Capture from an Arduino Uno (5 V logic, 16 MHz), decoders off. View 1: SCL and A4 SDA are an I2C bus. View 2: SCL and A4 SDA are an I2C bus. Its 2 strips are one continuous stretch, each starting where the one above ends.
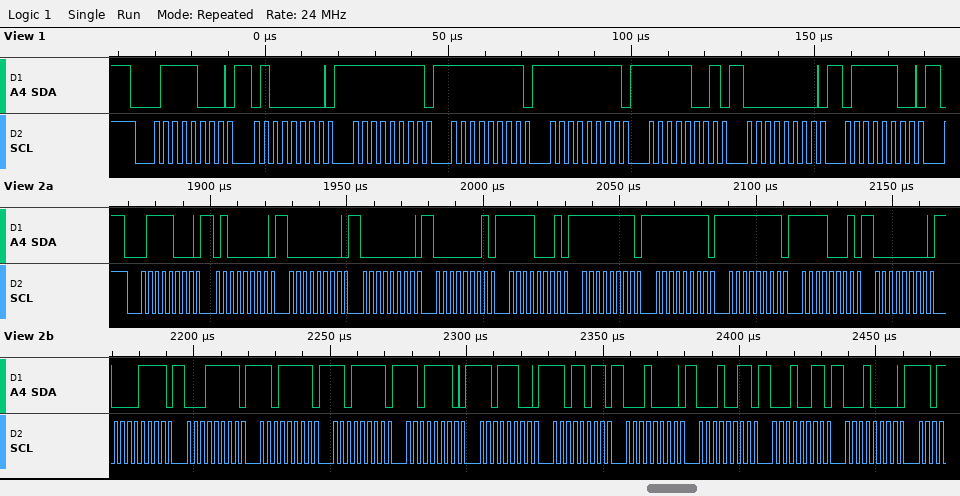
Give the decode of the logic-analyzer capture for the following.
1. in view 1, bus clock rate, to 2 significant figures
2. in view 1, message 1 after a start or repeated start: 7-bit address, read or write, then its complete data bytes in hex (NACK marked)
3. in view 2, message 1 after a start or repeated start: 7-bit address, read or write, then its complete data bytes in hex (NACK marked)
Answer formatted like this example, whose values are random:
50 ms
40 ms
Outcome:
400 kHz
0x3C write: 40 FF FF FF F9 00 7C
0x3C write: 40 00 00 01 F1 FF FF FF F1 00 0F 1F DF DF DE DC DB 10 13 13 10
